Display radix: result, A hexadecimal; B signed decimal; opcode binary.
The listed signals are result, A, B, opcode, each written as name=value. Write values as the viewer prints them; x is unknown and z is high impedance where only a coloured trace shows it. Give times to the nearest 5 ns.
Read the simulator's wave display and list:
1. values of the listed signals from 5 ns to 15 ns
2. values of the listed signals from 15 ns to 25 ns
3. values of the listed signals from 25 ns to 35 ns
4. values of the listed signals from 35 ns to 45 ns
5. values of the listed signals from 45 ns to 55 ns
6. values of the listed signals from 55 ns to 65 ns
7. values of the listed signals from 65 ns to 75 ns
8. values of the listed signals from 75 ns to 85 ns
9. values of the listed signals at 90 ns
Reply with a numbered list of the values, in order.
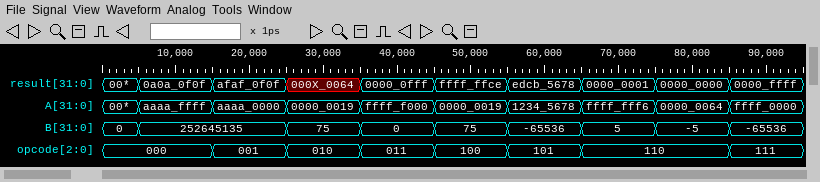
1. result=0a0a_0f0f, A=aaaa_ffff, B=252645135, opcode=000
2. result=afaf_0f0f, A=aaaa_0000, B=252645135, opcode=001
3. result=000X_0064, A=0000_0019, B=75, opcode=010
4. result=0000_0fff, A=ffff_f000, B=0, opcode=011
5. result=ffff_ffce, A=0000_0019, B=75, opcode=100
6. result=edcb_5678, A=1234_5678, B=-65536, opcode=101
7. result=0000_0001, A=ffff_fff6, B=5, opcode=110
8. result=0000_0000, A=0000_0064, B=-5, opcode=110
9. result=0000_ffff, A=ffff_0000, B=-65536, opcode=111
